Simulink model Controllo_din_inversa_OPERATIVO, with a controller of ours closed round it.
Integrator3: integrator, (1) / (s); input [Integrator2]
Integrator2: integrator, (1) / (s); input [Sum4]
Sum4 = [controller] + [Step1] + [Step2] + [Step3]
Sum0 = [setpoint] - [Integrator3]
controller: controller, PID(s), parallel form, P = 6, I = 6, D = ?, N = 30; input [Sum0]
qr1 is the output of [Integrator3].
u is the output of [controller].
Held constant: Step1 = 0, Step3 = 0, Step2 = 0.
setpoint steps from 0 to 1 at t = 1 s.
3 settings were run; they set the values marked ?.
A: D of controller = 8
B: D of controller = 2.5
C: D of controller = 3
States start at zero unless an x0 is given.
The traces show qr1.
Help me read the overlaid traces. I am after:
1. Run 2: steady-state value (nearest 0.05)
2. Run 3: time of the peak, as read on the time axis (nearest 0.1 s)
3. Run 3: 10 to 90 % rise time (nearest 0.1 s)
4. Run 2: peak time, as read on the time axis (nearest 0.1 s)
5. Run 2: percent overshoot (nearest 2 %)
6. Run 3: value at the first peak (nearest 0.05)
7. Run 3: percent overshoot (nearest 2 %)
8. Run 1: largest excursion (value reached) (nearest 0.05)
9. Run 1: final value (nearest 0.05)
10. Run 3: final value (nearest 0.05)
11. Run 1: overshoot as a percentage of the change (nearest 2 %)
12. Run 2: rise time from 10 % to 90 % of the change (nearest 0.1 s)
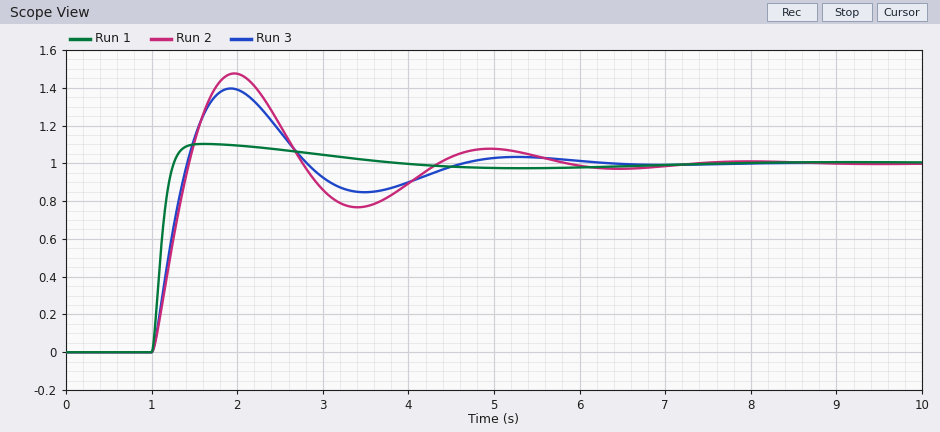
1.00
1.9 s
0.3 s
2.0 s
48 %
1.40
40 %
1.10
1.00
1.00
10 %
0.3 s
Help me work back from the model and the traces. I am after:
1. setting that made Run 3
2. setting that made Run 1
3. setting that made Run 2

C
A
B
